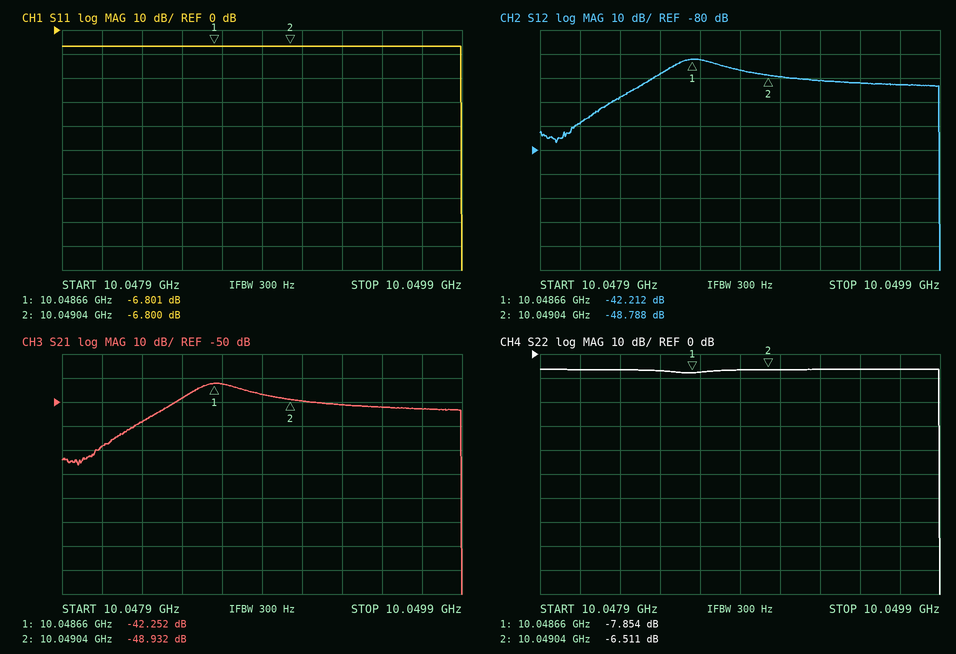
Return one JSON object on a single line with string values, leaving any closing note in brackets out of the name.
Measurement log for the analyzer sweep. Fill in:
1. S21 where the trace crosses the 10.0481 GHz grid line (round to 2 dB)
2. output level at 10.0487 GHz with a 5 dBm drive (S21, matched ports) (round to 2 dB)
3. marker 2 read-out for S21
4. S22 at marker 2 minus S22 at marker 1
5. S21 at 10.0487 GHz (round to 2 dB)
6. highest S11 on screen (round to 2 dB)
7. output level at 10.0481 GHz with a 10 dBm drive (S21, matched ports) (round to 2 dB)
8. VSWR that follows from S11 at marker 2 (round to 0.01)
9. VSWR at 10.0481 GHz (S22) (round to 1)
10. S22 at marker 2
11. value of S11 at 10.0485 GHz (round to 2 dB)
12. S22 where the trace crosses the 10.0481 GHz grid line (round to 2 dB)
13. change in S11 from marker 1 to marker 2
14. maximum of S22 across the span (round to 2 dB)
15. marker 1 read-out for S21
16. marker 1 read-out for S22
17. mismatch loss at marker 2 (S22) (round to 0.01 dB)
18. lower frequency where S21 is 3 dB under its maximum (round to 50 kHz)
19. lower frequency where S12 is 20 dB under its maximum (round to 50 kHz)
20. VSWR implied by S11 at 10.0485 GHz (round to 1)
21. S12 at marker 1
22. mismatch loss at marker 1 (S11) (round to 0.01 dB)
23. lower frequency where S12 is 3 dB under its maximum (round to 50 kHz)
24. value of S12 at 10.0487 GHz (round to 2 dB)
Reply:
{"S21 where the trace crosses the 10.0481 GHz grid line": "-68 dB", "output level at 10.0487 GHz with a 5 dBm drive (S21, matched ports)": "-38 dBm", "marker 2 read-out for S21": "-48.932 dB", "S22 at marker 2 minus S22 at marker 1": "1.343 dB", "S21 at 10.0487 GHz": "-42 dB", "highest S11 on screen": "-6 dB", "output level at 10.0481 GHz with a 10 dBm drive (S21, matched ports)": "-58 dBm", "VSWR that follows from S11 at marker 2": "2.68", "VSWR at 10.0481 GHz (S22)": "3", "S22 at marker 2": "-6.511 dB", "value of S11 at 10.0485 GHz": "-6 dB", "S22 where the trace crosses the 10.0481 GHz grid line": "-6 dB", "change in S11 from marker 1 to marker 2": "0.001 dB", "maximum of S22 across the span": "-6 dB", "marker 1 read-out for S21": "-42.252 dB", "marker 1 read-out for S22": "-7.854 dB", "mismatch loss at marker 2 (S22)": "1.10 dB", "lower frequency where S21 is 3 dB under its maximum": "10.04855 GHz", "lower frequency where S12 is 20 dB under its maximum": "10.04820 GHz", "VSWR implied by S11 at 10.0485 GHz": "3", "S12 at marker 1": "-42.212 dB", "mismatch loss at marker 1 (S11)": "1.02 dB", "lower frequency where S12 is 3 dB under its maximum": "10.04855 GHz", "value of S12 at 10.0487 GHz": "-42 dB"}
